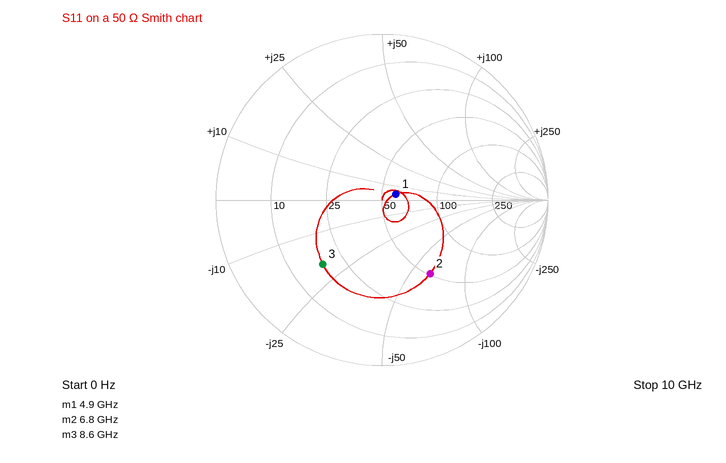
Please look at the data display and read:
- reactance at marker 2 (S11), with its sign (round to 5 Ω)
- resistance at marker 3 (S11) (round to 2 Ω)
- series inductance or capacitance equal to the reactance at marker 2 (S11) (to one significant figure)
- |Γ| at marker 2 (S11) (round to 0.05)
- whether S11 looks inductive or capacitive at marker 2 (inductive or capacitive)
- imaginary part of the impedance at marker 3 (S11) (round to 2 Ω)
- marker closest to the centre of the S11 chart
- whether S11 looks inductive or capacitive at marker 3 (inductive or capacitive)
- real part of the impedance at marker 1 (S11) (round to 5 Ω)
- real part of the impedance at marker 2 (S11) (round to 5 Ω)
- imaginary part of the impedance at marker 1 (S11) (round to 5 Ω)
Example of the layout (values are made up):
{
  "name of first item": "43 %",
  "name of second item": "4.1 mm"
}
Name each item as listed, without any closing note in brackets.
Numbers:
{
  "reactance at marker 2 (S11), with its sign": "-65 Ω",
  "resistance at marker 3 (S11)": "18 Ω",
  "series inductance or capacitance equal to the reactance at marker 2 (S11)": "400 fF",
  "|Γ| at marker 2 (S11)": "0.55",
  "whether S11 looks inductive or capacitive at marker 2": "capacitive",
  "imaginary part of the impedance at marker 3 (S11)": "-20 Ω",
  "marker closest to the centre of the S11 chart": "marker 1",
  "whether S11 looks inductive or capacitive at marker 3": "capacitive",
  "real part of the impedance at marker 1 (S11)": "60 Ω",
  "real part of the impedance at marker 2 (S11)": "50 Ω",
  "imaginary part of the impedance at marker 1 (S11)": "+5 Ω"
}
